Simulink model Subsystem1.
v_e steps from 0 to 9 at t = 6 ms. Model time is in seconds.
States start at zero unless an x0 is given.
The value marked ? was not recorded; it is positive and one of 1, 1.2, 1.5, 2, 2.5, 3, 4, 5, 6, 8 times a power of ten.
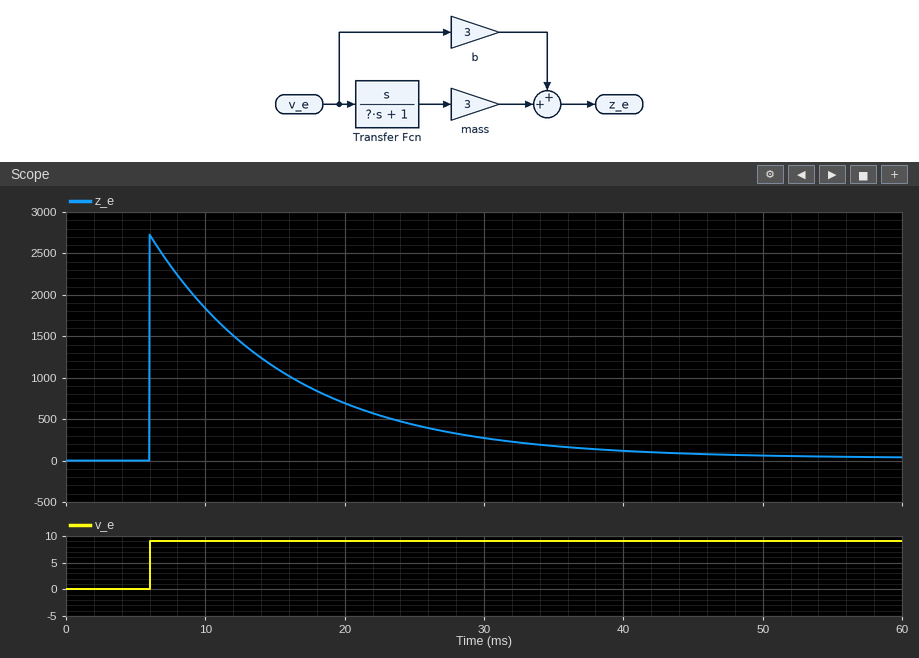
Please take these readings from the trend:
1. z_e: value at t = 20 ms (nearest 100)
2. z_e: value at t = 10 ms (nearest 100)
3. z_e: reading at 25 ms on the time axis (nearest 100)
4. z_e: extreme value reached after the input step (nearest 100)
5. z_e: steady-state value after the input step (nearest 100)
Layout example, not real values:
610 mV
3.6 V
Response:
700
1800
400
2700
0
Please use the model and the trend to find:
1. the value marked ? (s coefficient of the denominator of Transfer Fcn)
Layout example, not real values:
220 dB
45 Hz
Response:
0.01
